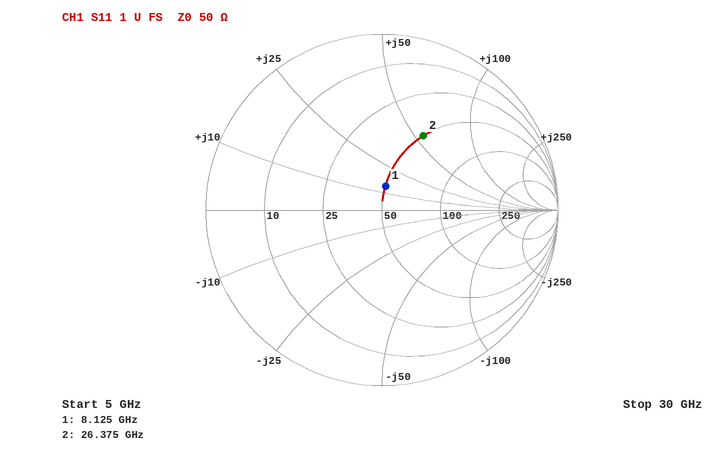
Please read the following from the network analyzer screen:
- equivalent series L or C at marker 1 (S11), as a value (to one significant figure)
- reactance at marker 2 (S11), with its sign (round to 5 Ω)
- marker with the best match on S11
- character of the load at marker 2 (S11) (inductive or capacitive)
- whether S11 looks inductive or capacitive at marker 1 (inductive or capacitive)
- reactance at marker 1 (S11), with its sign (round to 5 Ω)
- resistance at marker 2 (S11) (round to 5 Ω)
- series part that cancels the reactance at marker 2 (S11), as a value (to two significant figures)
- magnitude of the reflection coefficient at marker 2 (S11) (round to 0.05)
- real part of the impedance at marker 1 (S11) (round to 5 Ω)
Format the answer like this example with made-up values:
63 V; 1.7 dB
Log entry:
300 pH; +55 Ω; marker 1; inductive; inductive; +15 Ω; 50 Ω; 110 fF; 0.50; 50 Ω
